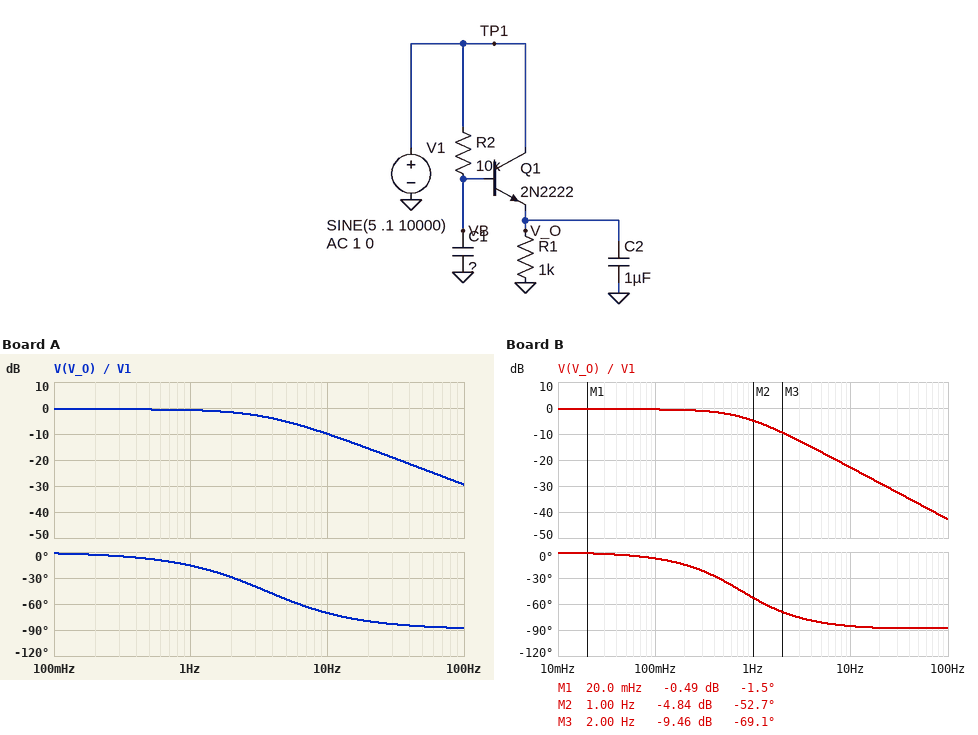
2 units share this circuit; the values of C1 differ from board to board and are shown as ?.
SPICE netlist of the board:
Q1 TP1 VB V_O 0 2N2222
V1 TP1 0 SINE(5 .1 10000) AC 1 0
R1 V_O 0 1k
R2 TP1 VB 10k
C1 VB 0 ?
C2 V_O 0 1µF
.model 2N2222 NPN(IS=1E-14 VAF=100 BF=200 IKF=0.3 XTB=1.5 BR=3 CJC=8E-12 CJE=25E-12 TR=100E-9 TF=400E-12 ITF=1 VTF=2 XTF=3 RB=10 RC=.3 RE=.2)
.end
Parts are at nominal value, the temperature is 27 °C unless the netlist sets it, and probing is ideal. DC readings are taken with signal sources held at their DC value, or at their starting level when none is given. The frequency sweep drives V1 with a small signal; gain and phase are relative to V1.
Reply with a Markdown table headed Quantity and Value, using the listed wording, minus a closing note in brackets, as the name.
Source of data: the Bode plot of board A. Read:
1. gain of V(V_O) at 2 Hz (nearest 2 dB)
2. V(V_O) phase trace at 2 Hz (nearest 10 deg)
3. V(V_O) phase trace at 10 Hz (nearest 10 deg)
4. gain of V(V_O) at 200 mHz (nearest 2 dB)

| Quantity | Value |
|---|---|
| gain of V(V_O) at 2 Hz | -2 dB |
| V(V_O) phase trace at 2 Hz | -30 deg |
| V(V_O) phase trace at 10 Hz | -70 deg |
| gain of V(V_O) at 200 mHz | 0 dB |
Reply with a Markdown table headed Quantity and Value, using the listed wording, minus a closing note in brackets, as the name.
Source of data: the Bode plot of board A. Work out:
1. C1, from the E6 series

| Quantity | Value |
|---|---|
| C1, from the E6 series | 4.7 µF |
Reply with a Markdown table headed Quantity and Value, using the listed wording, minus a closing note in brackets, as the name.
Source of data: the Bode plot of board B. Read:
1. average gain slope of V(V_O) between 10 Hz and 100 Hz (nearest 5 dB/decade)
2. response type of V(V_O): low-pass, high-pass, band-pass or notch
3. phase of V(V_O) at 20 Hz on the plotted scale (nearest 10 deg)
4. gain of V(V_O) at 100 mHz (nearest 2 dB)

| Quantity | Value |
|---|---|
| average gain slope of V(V_O) between 10 Hz and 100 Hz | -20 dB/decade |
| response type of V(V_O): low-pass, high-pass, band-pass or notch | low-pass |
| phase of V(V_O) at 20 Hz on the plotted scale | -90 deg |
| gain of V(V_O) at 100 mHz | 0 dB |
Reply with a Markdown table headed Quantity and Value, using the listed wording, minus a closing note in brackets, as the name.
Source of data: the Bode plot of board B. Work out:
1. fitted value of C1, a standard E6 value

| Quantity | Value |
|---|---|
| fitted value of C1, a standard E6 value | 22 µF |
